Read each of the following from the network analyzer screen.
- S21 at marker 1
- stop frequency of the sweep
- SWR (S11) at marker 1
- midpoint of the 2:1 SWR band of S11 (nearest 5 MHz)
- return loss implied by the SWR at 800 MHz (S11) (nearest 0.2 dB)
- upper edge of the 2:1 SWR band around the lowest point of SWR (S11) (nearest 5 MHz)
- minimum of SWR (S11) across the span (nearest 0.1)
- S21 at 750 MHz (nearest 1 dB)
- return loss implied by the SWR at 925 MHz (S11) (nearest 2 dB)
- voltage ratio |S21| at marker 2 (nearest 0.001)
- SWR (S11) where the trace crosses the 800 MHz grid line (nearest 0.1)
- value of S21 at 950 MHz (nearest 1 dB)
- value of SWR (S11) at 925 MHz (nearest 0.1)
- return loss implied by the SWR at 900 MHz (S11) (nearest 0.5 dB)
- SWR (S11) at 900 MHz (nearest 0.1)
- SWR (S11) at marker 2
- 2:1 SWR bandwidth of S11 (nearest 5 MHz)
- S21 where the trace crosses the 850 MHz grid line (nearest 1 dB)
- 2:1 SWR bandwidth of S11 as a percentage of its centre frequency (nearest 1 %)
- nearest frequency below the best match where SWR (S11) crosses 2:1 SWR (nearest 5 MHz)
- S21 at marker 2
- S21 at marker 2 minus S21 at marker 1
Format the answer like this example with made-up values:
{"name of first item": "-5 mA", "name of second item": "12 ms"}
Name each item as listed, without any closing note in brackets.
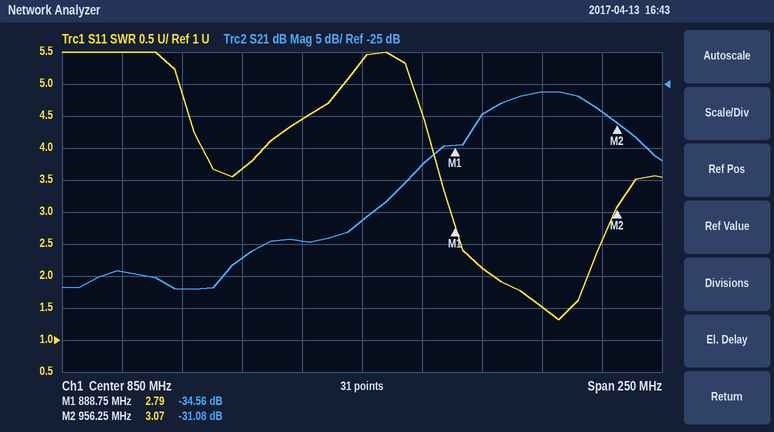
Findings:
{"S21 at marker 1": "-34.56 dB", "stop frequency of the sweep": "975 MHz", "SWR (S11) at marker 1": "2.79", "midpoint of the 2:1 SWR band of S11": "925 MHz", "return loss implied by the SWR at 800 MHz (S11)": "4.8 dB", "upper edge of the 2:1 SWR band around the lowest point of SWR (S11)": "945 MHz", "minimum of SWR (S11) across the span": "1.3", "S21 at 750 MHz": "-54 dB", "return loss implied by the SWR at 925 MHz (S11)": "14 dB", "voltage ratio |S21| at marker 2": "0.028", "SWR (S11) where the trace crosses the 800 MHz grid line": "3.7", "value of S21 at 950 MHz": "-29 dB", "value of SWR (S11) at 925 MHz": "1.5", "return loss implied by the SWR at 900 MHz (S11)": "9.0 dB", "SWR (S11) at 900 MHz": "2.1", "SWR (S11) at marker 2": "3.07", "2:1 SWR bandwidth of S11": "40 MHz", "S21 where the trace crosses the 850 MHz grid line": "-46 dB", "2:1 SWR bandwidth of S11 as a percentage of its centre frequency": "4 %", "nearest frequency below the best match where SWR (S11) crosses 2:1 SWR": "905 MHz", "S21 at marker 2": "-31.08 dB", "S21 at marker 2 minus S21 at marker 1": "3.48 dB"}
